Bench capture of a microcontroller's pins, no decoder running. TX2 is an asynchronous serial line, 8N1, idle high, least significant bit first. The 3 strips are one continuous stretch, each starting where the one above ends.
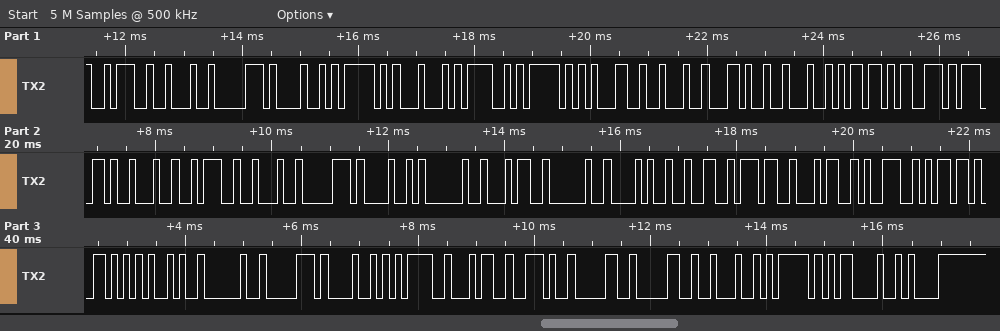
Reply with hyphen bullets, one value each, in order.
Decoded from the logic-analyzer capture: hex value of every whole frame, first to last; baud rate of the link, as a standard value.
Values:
- 0x3A 0x22 0x70 0x48 0x5F 0x44 0x4F 0x5F 0x31 0x22 0x2C 0x22 0x6D 0x73 0x67 0x22 0x3A 0x22 0x70 0x48 0x20 0x34 0x20 0x28 0x32 0x37 0x34 0x39 0x6D 0x56 0x29 0x20 0x70 0x48 0x3D 0x34 0x2E 0x30 0x30 0x22 0x7D 0x0D 0x0A
- 9600 baud
